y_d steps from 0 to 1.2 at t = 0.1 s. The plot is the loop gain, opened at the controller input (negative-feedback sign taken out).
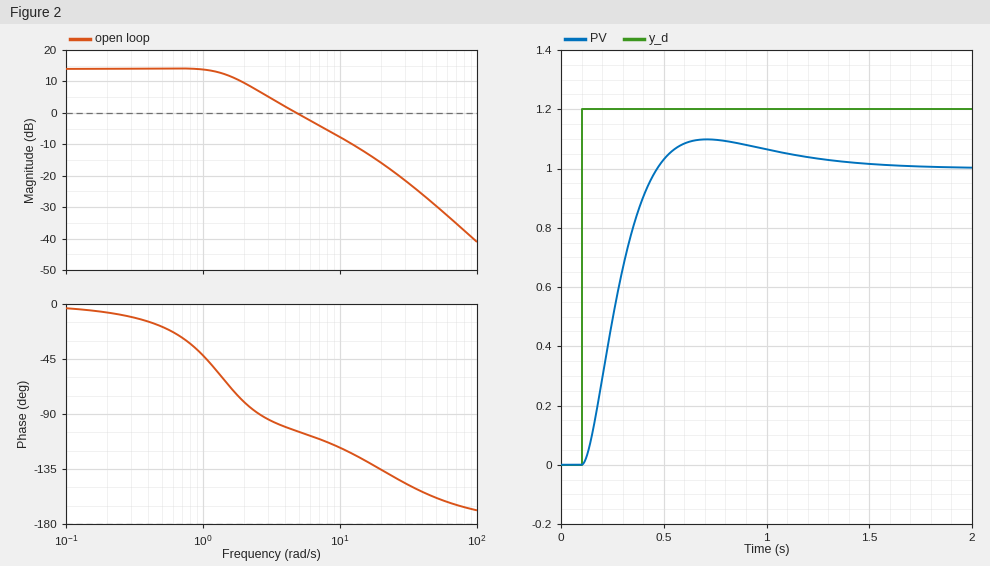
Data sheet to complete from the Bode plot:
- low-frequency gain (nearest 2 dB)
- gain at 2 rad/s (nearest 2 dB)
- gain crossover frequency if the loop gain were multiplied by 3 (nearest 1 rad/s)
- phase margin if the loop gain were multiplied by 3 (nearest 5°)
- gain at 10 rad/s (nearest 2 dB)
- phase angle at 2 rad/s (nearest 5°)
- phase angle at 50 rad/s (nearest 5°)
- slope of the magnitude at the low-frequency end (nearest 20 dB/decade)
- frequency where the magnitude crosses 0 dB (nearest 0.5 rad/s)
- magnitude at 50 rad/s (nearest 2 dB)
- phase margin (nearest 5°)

14 dB
10 dB
12 rad/s
60°
-8 dB
-80°
-160°
0 dB/decade
5.0 rad/s
-30 dB
75°
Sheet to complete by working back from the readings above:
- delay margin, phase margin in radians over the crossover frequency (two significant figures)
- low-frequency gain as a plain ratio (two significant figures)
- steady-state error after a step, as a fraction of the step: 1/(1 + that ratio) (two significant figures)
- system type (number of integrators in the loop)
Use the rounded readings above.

0.26 s
5.0
0.17
0
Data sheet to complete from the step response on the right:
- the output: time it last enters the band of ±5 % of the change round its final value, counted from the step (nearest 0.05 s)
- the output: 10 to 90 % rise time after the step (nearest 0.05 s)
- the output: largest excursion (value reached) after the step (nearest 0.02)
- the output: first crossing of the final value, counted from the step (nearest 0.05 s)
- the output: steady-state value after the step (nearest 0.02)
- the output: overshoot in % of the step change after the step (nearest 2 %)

1.00 s
0.25 s
1.10
0.35 s
1.00
10 %
